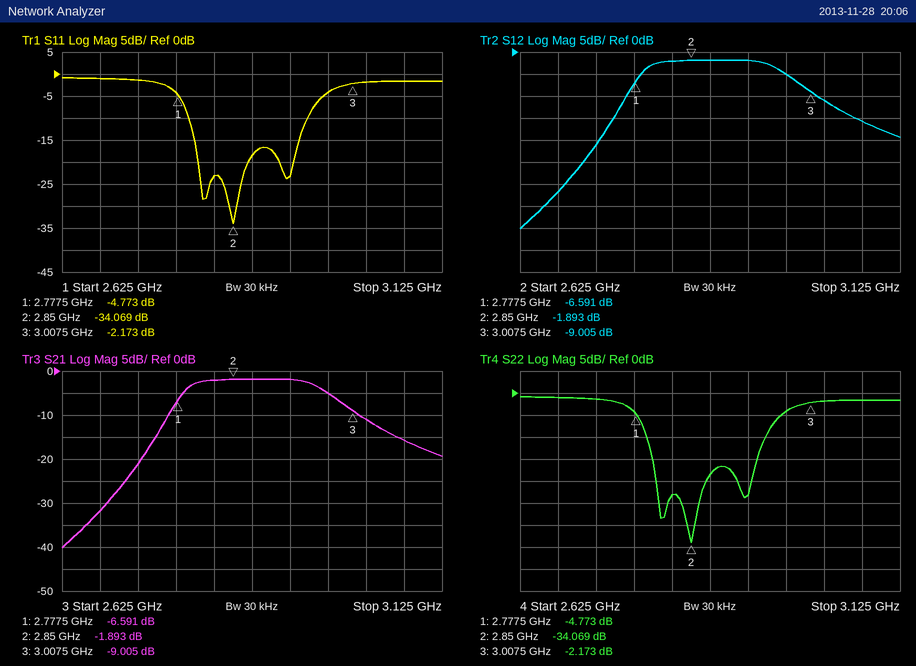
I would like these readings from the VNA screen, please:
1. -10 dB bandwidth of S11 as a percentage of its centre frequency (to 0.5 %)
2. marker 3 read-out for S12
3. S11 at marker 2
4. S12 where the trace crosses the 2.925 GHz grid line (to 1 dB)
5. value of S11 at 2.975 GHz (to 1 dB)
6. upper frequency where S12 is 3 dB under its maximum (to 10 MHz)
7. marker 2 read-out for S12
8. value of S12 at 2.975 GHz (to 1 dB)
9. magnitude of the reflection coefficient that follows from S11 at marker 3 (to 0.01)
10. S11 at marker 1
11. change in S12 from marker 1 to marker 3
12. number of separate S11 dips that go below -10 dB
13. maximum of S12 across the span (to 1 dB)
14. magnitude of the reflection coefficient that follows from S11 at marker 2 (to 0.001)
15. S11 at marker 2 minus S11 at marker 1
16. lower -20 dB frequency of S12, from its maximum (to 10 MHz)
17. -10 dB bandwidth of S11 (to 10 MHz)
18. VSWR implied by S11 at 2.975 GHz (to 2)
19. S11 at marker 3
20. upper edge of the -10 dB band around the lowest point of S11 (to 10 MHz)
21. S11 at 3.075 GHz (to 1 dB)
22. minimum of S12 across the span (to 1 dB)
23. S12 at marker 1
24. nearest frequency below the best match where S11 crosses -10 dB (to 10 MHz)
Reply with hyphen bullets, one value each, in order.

- 5.5 %
- -9.005 dB
- -34.069 dB
- -2 dB
- -4 dB
- 2.97 GHz
- -1.893 dB
- -5 dB
- 0.78
- -4.773 dB
- -2.414 dB
- 3
- -2 dB
- 0.020
- -29.296 dB
- 2.72 GHz
- 160 MHz
- 4
- -2.173 dB
- 2.95 GHz
- -2 dB
- -40 dB
- -6.591 dB
- 2.79 GHz
